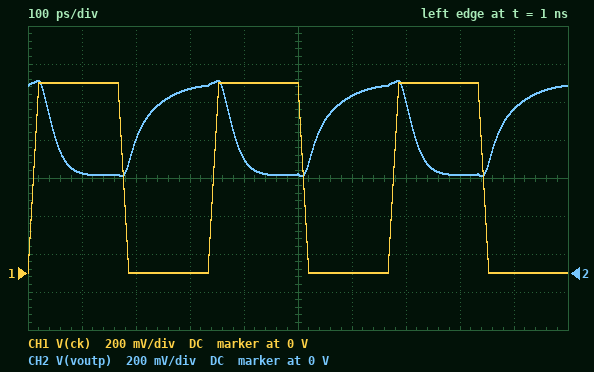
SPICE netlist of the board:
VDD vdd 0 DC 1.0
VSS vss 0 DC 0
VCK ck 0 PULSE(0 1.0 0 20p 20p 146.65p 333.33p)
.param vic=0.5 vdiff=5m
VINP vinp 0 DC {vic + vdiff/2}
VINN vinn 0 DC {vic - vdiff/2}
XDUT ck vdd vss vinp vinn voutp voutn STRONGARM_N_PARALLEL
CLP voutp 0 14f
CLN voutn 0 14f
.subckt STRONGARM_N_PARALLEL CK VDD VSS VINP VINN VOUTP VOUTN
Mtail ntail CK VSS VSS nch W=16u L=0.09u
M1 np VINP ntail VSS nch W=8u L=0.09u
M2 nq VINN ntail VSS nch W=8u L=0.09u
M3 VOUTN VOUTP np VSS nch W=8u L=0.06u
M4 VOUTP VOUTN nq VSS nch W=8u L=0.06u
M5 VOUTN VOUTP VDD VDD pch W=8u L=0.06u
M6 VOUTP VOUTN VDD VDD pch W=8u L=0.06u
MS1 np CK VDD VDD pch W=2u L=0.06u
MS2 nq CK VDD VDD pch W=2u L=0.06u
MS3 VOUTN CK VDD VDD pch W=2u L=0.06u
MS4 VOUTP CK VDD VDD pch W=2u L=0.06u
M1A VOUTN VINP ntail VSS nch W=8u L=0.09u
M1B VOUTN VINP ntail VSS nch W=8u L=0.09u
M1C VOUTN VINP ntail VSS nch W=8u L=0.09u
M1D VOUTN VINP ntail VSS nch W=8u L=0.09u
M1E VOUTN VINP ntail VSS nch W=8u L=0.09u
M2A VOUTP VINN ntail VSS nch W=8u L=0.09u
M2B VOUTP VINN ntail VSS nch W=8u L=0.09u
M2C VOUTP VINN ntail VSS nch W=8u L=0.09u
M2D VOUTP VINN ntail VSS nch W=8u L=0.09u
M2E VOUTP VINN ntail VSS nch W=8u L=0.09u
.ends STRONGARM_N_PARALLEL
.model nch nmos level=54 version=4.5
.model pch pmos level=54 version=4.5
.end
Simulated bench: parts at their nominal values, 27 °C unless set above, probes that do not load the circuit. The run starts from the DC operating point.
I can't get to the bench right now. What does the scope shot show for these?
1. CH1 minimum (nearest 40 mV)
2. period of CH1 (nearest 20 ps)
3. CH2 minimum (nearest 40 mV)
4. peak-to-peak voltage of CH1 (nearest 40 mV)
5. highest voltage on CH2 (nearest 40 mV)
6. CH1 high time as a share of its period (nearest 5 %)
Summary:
0 V
340 ps
520 mV
1.00 V
1.00 V
50 %
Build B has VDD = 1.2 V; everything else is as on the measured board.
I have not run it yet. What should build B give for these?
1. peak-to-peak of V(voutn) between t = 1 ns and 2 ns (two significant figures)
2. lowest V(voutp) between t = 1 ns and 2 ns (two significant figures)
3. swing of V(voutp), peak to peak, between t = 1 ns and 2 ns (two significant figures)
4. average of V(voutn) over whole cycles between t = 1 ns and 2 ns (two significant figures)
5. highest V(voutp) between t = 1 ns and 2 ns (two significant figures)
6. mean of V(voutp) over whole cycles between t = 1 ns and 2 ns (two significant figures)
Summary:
630 mV
690 mV
520 mV
880 mV
1.2 V
950 mV
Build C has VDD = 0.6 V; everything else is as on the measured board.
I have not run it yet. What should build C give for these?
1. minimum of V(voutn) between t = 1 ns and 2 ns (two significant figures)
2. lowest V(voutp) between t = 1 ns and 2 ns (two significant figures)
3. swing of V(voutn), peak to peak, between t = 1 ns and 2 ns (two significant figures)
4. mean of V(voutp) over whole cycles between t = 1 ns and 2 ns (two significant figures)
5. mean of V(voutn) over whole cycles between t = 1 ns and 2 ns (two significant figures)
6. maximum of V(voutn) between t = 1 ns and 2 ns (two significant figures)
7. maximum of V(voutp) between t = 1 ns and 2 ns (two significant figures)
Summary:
110 mV
120 mV
360 mV
280 mV
260 mV
470 mV
490 mV
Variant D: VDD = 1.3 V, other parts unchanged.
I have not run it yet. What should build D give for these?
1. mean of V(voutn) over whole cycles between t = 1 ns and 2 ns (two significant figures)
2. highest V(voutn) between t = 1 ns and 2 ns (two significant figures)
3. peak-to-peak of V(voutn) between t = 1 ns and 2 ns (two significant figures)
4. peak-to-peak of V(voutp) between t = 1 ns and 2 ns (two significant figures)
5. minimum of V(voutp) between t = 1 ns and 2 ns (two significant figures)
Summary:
990 mV
1.3 V
630 mV
520 mV
790 mV
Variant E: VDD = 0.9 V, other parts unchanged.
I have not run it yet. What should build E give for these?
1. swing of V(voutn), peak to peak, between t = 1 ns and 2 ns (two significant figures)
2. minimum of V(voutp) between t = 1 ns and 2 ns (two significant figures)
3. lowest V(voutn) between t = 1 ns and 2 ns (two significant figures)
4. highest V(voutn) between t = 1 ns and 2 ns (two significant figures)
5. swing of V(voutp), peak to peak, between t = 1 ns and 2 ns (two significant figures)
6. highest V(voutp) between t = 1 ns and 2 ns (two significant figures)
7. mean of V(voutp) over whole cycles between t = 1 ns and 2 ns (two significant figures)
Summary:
560 mV
420 mV
290 mV
850 mV
480 mV
900 mV
650 mV
